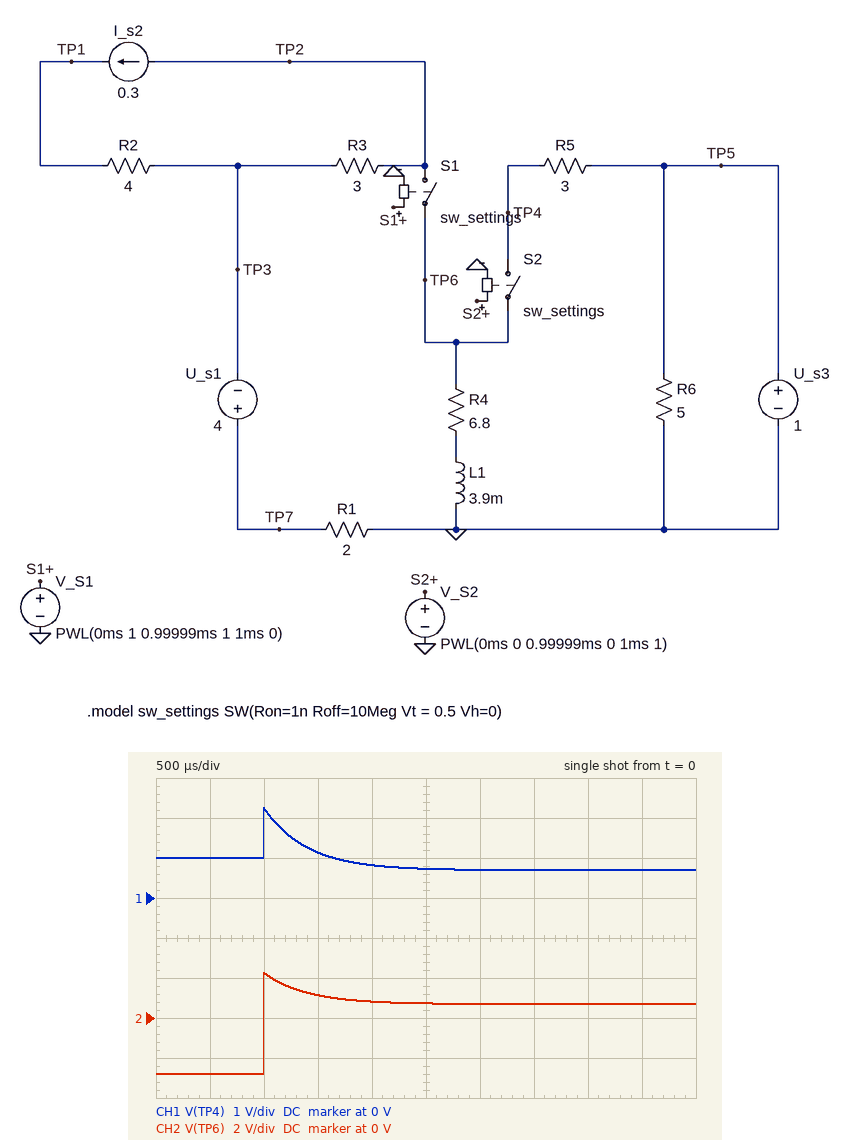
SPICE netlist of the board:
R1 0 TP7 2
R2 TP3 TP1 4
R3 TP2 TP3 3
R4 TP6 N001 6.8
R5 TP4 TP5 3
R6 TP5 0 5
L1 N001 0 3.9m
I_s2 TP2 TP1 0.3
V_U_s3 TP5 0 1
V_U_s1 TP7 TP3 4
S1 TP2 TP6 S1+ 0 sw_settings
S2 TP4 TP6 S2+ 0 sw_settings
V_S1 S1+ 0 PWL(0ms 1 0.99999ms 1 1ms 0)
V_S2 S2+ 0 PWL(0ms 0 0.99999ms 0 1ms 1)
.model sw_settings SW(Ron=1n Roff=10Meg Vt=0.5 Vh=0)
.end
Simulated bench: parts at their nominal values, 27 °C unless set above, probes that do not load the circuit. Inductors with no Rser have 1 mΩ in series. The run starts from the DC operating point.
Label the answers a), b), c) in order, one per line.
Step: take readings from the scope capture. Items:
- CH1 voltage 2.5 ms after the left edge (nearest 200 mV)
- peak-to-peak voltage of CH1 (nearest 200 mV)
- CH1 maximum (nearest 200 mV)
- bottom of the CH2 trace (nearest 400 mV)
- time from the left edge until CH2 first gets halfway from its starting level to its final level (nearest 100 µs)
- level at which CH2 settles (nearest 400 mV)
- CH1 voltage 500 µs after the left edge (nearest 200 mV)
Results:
a) 800 mV
b) 1.6 V
c) 2.2 V
d) -2.8 V
e) 1.0 ms
f) 800 mV
g) 1.0 V
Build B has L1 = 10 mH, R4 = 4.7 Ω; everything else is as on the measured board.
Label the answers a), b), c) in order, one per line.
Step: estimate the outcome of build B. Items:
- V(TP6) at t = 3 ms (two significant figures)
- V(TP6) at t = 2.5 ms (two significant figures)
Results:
a) 1.0 V
b) 1.2 V
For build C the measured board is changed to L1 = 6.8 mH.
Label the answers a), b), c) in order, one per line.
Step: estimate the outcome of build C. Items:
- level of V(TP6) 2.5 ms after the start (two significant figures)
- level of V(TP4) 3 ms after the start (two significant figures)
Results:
a) 870 mV
b) 780 mV
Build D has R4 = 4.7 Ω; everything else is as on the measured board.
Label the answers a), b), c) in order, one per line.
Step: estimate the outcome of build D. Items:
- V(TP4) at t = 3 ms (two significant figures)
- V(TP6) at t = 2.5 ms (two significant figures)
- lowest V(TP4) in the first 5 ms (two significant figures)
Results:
a) 650 mV
b) 710 mV
c) 610 mV
